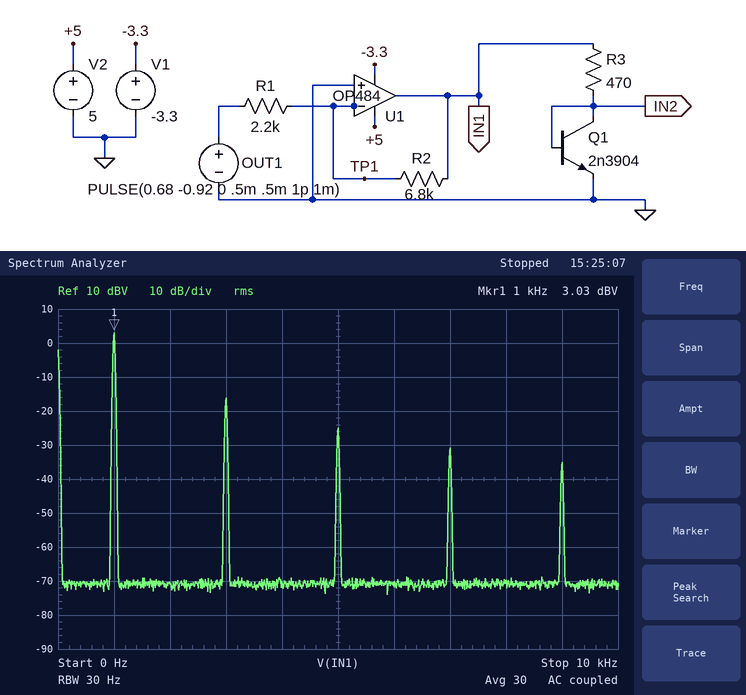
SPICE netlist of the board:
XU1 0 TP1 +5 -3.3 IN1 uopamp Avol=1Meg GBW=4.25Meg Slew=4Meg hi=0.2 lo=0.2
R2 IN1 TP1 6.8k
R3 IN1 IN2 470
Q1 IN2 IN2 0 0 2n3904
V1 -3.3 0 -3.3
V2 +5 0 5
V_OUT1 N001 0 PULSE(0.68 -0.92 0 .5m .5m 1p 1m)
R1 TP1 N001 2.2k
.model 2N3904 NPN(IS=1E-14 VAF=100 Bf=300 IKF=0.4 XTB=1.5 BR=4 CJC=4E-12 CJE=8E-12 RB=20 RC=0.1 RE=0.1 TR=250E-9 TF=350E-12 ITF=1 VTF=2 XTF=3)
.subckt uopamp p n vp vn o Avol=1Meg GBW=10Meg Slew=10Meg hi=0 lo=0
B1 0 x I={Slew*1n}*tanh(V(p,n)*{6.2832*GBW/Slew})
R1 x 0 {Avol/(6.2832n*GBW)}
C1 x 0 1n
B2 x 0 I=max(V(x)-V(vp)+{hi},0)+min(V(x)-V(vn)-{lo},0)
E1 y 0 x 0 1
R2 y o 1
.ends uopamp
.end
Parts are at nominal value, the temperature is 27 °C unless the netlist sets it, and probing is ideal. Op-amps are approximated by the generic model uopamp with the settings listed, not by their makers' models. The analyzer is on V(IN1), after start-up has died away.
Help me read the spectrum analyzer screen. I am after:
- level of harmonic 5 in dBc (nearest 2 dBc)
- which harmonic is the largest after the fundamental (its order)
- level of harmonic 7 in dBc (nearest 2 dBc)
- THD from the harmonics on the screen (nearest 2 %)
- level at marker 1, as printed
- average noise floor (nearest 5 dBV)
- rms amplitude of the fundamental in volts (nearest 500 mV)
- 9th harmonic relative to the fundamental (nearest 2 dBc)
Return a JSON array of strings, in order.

["-28 dBc", "3", "-34 dBc", "12 %", "3.03 dBV", "-70 dBV", "1.5 V", "-38 dBc"]
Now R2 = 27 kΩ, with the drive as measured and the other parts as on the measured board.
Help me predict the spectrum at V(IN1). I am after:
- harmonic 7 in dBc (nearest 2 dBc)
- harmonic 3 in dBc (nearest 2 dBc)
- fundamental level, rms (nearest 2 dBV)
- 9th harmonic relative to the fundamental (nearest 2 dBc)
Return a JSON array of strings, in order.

["-32 dBc", "-16 dBc", "10 dBV", "-42 dBc"]
